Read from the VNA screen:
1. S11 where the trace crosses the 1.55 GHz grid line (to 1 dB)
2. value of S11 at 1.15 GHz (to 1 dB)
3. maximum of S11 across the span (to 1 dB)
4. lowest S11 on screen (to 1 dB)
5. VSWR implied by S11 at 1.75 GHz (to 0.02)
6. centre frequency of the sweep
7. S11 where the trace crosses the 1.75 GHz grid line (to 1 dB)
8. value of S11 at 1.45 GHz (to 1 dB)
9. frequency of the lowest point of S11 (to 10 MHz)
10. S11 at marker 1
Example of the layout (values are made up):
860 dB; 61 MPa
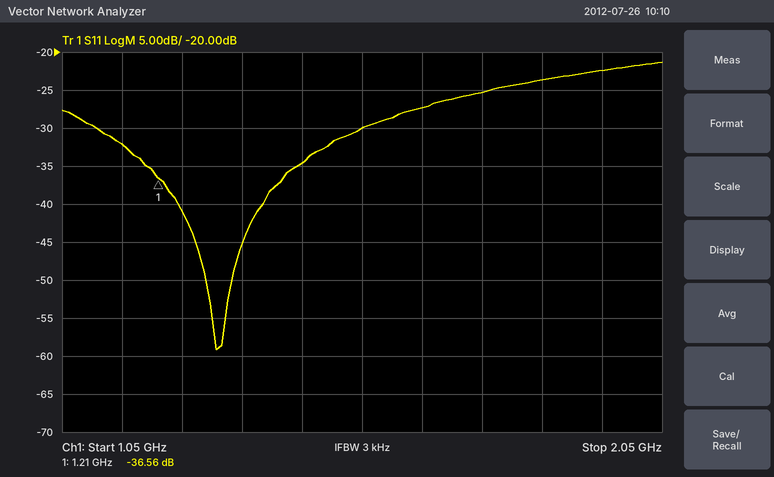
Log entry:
-30 dB; -32 dB; -21 dB; -59 dB; 1.12; 1.55 GHz; -25 dB; -35 dB; 1.31 GHz; -36.56 dB
